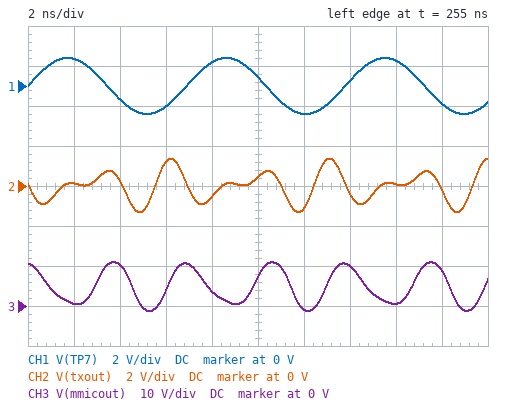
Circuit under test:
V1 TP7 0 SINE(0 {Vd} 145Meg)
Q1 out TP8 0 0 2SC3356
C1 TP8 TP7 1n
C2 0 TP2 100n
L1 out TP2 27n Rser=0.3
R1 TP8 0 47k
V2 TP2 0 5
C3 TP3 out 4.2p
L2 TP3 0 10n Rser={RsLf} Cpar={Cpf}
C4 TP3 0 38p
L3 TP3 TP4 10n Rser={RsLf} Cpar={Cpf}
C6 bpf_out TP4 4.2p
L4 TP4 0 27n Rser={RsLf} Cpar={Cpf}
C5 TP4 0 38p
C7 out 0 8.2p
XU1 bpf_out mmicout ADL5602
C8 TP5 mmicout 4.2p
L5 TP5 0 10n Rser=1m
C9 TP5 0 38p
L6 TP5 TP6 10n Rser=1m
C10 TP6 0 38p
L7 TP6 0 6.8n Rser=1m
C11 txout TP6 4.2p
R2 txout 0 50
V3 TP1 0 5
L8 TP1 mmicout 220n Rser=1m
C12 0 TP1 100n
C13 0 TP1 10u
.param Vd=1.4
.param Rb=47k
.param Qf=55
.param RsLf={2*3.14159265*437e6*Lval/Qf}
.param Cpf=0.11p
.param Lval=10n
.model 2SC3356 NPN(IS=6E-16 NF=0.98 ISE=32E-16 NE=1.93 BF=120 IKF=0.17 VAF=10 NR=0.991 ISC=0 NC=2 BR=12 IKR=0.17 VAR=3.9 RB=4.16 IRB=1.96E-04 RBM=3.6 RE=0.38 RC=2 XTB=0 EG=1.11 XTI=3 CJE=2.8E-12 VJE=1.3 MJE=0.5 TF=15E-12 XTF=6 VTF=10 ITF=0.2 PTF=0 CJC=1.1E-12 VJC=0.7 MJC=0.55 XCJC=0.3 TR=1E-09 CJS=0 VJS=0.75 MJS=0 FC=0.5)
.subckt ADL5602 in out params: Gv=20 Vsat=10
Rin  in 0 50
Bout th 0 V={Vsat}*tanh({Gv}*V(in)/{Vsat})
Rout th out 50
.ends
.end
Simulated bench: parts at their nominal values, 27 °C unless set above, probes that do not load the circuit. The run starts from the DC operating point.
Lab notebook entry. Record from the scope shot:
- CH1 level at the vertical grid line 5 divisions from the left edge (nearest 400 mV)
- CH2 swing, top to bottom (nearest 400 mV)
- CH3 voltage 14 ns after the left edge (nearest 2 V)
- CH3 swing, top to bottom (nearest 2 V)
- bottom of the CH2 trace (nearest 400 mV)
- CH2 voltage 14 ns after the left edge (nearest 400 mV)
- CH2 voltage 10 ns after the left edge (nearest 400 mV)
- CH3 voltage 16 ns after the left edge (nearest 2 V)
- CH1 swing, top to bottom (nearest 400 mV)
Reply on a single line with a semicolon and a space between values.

400 mV; 2.8 V; 10 V; 12 V; -1.2 V; -400 mV; 400 mV; 0 V; 2.8 V
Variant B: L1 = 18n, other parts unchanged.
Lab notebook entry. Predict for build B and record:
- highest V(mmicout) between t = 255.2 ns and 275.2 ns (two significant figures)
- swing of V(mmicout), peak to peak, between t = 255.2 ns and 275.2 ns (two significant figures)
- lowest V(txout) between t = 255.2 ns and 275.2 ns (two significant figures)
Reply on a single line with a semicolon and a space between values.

13 V; 16 V; -2.4 V
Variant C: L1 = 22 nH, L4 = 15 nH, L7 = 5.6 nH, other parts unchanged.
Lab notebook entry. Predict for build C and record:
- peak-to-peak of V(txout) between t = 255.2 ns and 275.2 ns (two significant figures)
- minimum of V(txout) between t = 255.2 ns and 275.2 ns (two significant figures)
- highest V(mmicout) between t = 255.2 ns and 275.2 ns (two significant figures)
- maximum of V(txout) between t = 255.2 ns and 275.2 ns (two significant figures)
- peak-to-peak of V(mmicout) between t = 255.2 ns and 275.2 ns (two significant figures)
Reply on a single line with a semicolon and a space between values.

4.9 V; -2.4 V; 14 V; 2.5 V; 16 V
